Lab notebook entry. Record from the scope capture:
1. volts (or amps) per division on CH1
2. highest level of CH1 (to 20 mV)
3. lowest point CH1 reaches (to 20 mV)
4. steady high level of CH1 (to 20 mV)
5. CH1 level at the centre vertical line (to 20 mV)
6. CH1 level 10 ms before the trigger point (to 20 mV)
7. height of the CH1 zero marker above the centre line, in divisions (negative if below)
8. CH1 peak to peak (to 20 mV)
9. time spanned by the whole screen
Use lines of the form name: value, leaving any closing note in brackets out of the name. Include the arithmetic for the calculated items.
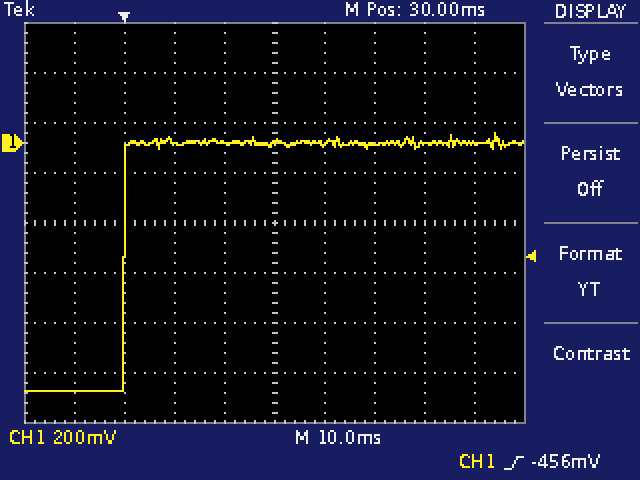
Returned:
volts (or amps) per division on CH1: 200 mV
highest level of CH1: 40 mV
lowest point CH1 reaches: -1.00 V
steady high level of CH1: 0 mV
CH1 level at the centre vertical line: 0 mV
CH1 level 10 ms before the trigger point: -1.00 V
height of the CH1 zero marker above the centre line, in divisions: +1.6 div
CH1 peak to peak: 40 mV − (-1.00 V) = 1.04 V
time spanned by the whole screen: 100 ms
